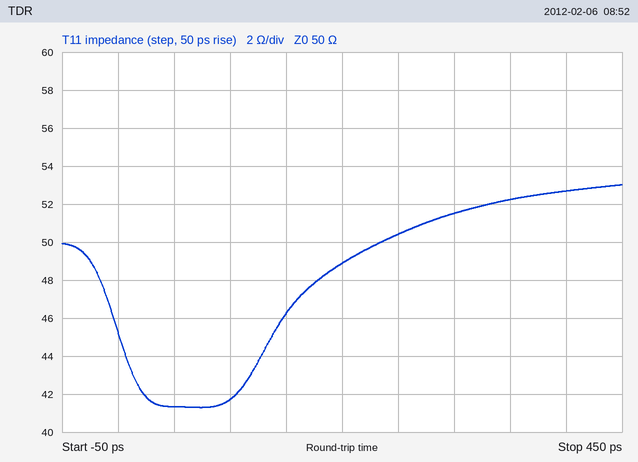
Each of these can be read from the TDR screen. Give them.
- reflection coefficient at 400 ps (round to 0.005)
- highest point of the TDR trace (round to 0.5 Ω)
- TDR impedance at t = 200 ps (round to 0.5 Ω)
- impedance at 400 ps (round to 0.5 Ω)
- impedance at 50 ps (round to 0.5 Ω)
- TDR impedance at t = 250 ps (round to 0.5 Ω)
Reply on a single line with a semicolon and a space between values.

+0.025; 53.0 Ω; 49.0 Ω; 52.5 Ω; 41.5 Ω; 50.5 Ω
